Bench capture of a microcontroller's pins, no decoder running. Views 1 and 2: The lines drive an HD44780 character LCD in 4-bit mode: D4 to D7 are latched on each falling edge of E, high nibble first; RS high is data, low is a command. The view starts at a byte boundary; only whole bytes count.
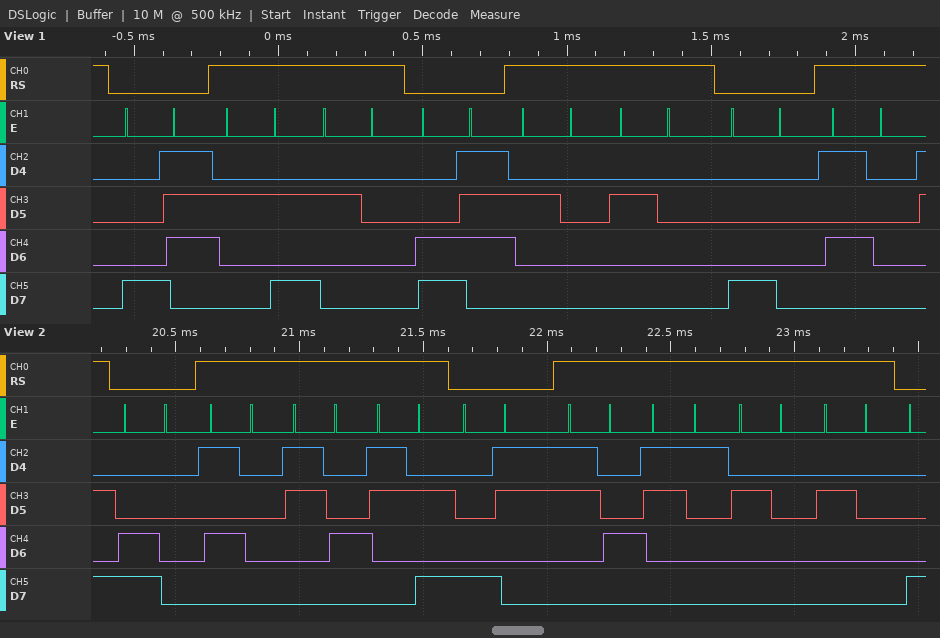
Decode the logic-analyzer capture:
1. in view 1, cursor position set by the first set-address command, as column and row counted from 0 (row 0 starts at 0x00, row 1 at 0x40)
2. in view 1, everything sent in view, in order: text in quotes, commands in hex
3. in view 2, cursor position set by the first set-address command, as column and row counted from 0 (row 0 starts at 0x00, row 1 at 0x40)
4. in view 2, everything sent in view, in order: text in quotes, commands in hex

column 7, row 0
0x87 "* " 0xC7 "  " 0x80 "P"
column 0, row 1
0xC0 "P4:" 0x83 "41  "
